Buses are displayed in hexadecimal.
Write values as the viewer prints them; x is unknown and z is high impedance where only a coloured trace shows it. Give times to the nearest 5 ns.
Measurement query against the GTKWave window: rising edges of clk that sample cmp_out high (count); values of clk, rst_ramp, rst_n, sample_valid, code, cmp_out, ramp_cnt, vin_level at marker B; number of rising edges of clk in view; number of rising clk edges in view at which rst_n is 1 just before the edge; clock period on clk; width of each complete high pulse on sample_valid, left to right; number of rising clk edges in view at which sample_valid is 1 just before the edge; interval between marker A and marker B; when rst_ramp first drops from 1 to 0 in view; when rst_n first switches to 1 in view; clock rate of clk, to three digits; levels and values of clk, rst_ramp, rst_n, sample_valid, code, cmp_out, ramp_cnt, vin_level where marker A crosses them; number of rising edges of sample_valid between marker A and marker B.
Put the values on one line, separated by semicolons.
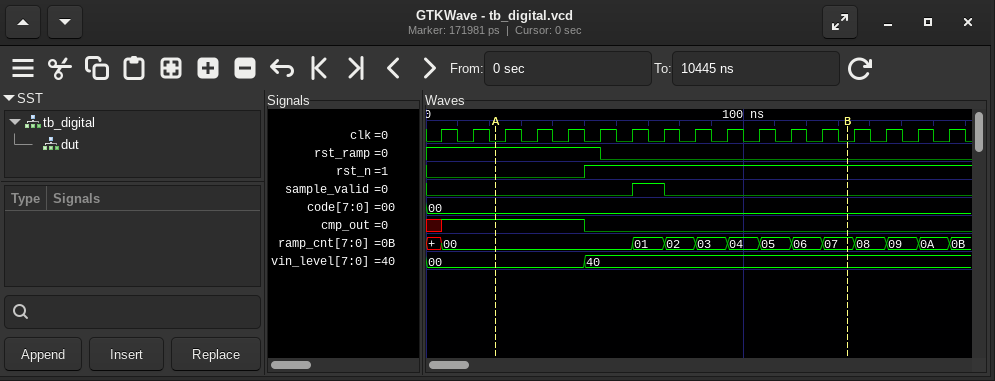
4; clk=0, rst_ramp=0, rst_n=1, sample_valid=0, code=00, cmp_out=0, ramp_cnt=07, vin_level=40; 17; 12; 10 ns; 10 ns; 1; 110 ns; 55 ns; 50 ns; 100 MHz; clk=0, rst_ramp=1, rst_n=0, sample_valid=0, code=00, cmp_out=1, ramp_cnt=00, vin_level=00; 1
